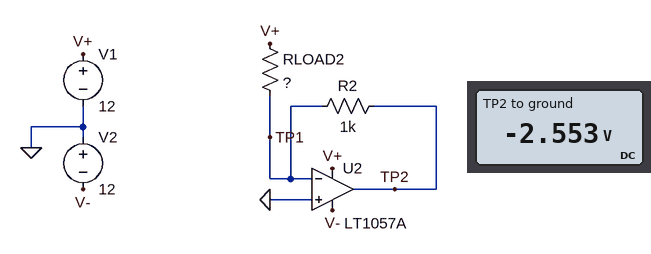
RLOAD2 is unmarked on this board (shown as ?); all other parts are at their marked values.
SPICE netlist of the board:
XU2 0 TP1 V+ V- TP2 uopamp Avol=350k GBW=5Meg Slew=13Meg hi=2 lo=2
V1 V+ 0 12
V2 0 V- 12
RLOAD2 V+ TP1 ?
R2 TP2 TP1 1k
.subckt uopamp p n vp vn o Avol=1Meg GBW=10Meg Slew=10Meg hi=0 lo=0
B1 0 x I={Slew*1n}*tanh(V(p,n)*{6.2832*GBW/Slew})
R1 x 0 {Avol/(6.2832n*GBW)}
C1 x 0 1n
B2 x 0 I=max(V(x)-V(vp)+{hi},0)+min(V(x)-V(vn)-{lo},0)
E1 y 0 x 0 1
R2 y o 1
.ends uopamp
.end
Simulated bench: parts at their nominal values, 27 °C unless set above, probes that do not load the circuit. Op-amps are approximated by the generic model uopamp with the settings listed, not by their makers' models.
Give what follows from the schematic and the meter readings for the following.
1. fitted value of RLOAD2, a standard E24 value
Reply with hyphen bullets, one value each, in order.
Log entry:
- 4.7 kΩ
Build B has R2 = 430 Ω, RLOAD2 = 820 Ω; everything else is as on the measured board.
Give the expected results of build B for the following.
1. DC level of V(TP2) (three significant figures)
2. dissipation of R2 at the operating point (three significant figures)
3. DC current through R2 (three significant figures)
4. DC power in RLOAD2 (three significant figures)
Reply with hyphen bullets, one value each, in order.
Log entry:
- -6.29 V
- 92.1 mW
- 14.6 mA
- 176 mW
